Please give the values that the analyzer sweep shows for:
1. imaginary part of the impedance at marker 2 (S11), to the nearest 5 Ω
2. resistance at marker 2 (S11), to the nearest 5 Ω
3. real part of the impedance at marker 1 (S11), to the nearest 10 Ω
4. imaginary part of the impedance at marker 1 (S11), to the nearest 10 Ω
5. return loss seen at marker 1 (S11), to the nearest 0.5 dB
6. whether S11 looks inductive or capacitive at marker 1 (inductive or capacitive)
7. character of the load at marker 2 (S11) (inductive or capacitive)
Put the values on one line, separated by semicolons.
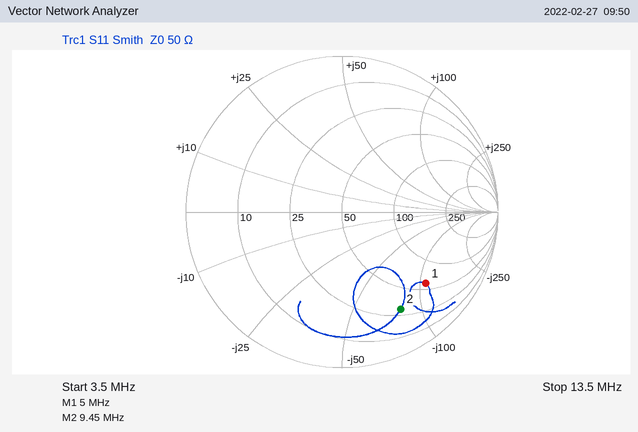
-80 Ω; 30 Ω; 60 Ω; -110 Ω; 3.0 dB; capacitive; capacitive
